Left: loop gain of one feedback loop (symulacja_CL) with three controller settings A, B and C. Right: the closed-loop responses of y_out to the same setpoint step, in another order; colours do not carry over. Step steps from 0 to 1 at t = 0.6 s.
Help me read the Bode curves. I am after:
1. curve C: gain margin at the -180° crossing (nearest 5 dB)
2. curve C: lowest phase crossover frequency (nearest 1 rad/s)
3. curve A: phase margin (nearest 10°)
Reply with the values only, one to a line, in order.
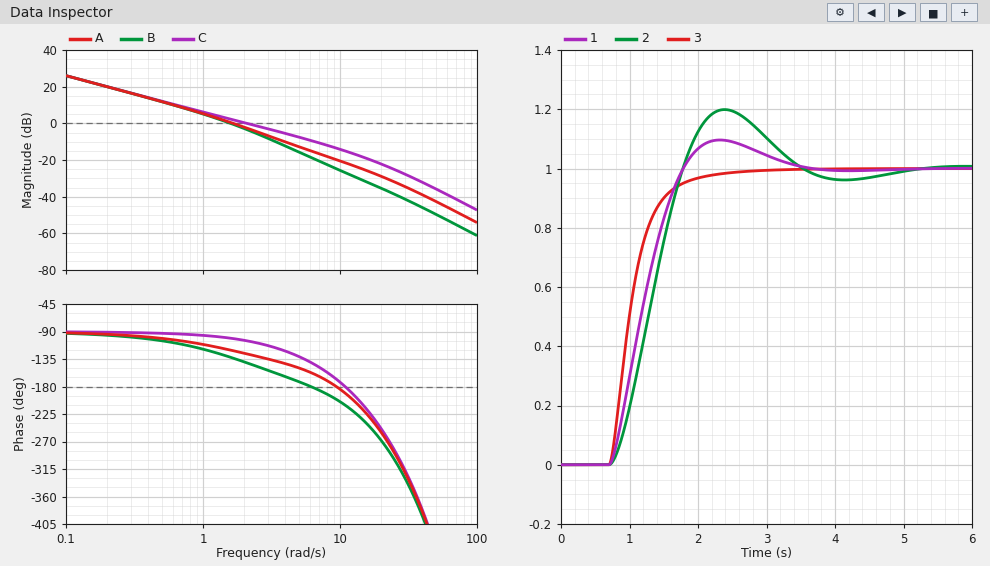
15 dB
11 rad/s
60°
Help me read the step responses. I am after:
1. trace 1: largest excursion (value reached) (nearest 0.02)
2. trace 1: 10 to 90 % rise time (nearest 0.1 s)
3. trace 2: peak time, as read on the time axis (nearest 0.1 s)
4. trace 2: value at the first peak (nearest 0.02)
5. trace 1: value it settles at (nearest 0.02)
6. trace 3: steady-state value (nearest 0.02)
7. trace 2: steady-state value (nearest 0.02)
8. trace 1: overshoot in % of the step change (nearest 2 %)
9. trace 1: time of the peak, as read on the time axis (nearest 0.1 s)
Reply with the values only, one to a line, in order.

1.10
0.8 s
2.4 s
1.20
1.00
1.00
1.00
10 %
2.3 s
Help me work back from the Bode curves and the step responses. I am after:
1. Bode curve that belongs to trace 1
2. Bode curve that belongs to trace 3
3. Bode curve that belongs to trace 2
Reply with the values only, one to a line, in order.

A
C
B
